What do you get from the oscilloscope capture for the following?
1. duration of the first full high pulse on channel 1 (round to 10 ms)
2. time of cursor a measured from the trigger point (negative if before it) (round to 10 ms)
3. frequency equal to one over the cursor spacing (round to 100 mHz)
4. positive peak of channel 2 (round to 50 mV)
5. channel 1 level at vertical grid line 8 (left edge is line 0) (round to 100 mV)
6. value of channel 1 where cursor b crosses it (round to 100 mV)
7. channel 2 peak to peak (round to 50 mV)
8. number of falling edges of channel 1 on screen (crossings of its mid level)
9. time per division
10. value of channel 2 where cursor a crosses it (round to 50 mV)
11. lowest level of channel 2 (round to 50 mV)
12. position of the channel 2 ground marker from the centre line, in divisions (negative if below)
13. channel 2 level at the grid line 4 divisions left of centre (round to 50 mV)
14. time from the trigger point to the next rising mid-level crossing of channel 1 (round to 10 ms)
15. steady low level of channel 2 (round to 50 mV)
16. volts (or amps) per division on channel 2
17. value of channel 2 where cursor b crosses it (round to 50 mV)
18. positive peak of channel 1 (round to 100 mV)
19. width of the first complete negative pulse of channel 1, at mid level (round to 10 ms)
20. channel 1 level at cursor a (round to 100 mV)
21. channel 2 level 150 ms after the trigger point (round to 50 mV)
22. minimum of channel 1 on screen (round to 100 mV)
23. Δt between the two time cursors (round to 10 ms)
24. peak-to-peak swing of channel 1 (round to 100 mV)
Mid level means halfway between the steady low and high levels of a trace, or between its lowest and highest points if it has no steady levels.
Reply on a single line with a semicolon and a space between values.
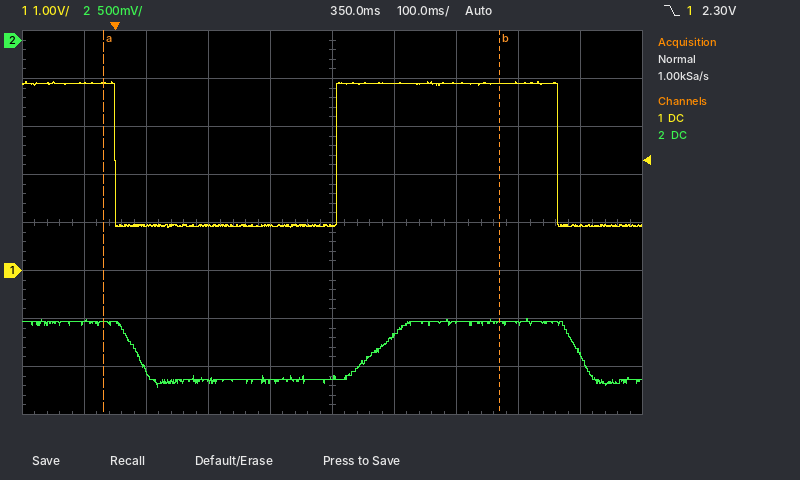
360 ms; -20 ms; 1.6 Hz; -2.90 V; 3.9 V; 3.9 V; 700 mV; 2; 100 ms; -2.95 V; -3.60 V; +3.8 div; -2.95 V; 360 ms; -3.55 V; 500 mV; -2.95 V; 3.9 V; 360 ms; 3.9 V; -3.55 V; 900 mV; 640 ms; 3.0 V
